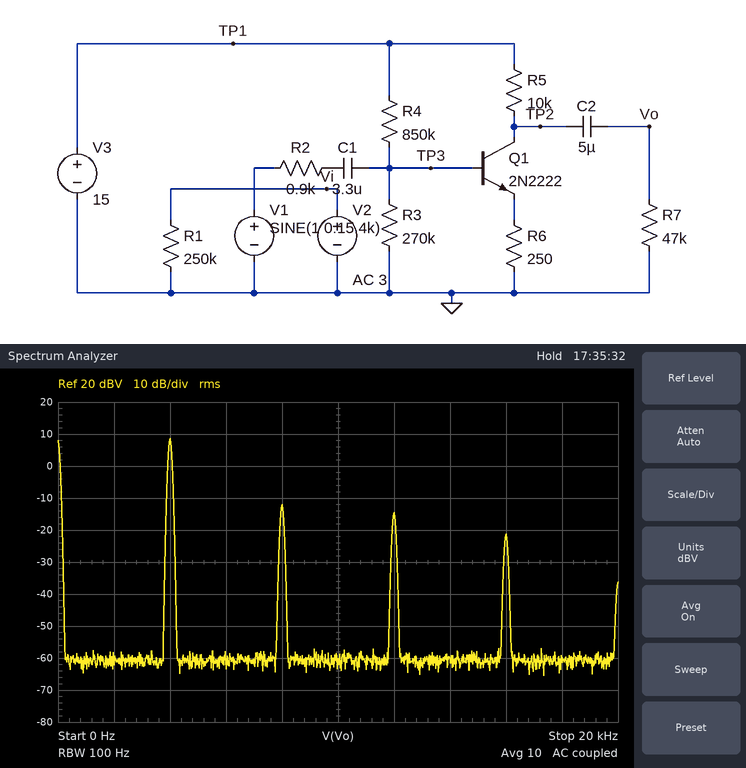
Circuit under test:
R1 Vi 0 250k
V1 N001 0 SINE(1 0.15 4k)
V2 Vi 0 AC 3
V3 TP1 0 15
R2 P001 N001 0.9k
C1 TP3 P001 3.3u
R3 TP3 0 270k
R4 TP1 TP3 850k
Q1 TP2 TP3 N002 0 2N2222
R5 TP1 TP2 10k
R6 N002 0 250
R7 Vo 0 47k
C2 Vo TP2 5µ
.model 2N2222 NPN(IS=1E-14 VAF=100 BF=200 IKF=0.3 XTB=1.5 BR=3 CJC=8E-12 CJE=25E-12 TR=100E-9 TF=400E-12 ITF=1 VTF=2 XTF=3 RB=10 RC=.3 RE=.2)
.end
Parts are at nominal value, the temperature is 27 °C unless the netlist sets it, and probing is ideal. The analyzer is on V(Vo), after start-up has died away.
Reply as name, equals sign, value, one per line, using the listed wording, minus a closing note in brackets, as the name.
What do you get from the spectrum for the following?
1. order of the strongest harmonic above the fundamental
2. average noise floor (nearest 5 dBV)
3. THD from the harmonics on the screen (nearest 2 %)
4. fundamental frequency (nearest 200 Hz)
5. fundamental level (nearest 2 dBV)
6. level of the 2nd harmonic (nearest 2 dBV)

order of the strongest harmonic above the fundamental = 2
average noise floor = -60 dBV
THD from the harmonics on the screen = 12 %
fundamental frequency = 4.0 kHz
fundamental level = 8 dBV
level of the 2nd harmonic = -12 dBV
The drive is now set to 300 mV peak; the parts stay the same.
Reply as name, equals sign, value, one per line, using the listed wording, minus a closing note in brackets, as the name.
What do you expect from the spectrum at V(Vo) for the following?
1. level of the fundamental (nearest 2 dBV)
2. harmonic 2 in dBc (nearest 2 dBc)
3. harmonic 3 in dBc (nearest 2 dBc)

level of the fundamental = 14 dBV
harmonic 2 in dBc = -36 dBc
harmonic 3 in dBc = -20 dBc
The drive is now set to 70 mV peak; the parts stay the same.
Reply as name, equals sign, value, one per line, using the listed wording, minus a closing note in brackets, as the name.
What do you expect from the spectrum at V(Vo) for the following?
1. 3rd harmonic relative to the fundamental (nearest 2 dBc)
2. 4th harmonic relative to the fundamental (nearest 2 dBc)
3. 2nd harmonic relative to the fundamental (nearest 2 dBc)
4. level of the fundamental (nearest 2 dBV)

3rd harmonic relative to the fundamental = -22 dBc
4th harmonic relative to the fundamental = -36 dBc
2nd harmonic relative to the fundamental = -16 dBc
level of the fundamental = 2 dBV
